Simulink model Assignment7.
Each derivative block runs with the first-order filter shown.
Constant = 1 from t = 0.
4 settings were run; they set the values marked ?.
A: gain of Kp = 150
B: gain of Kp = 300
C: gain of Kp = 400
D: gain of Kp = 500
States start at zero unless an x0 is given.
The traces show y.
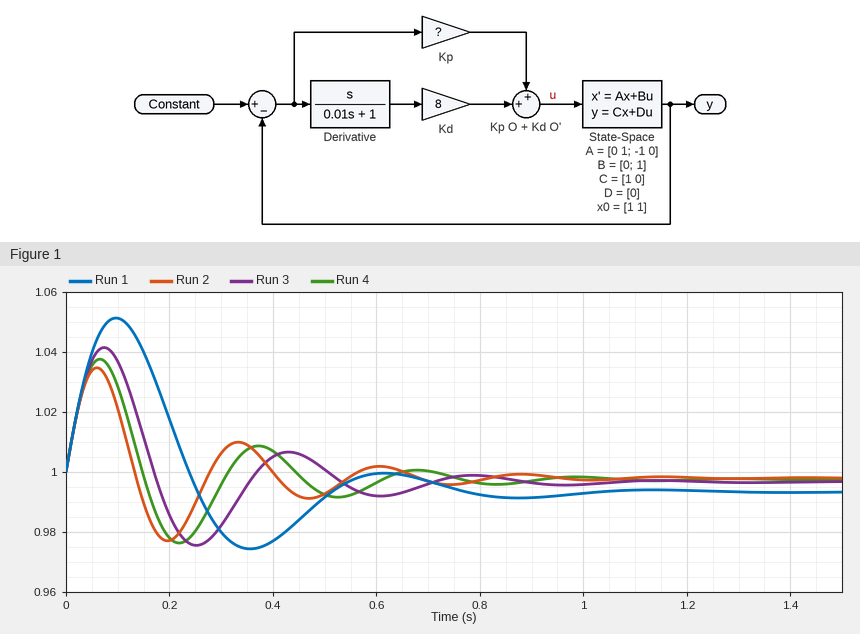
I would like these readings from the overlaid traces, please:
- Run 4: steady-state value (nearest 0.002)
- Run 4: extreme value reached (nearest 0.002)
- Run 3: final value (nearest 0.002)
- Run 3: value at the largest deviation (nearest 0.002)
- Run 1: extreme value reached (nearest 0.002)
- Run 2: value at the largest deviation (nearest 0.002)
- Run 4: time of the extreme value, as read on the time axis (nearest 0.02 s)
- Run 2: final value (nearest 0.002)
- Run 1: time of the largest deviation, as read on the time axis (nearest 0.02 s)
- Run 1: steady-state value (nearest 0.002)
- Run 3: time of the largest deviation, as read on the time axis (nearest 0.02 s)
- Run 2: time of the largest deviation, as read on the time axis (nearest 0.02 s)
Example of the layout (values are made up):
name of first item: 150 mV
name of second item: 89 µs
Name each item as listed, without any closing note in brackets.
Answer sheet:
Run 4: steady-state value: 0.998
Run 4: extreme value reached: 1.038
Run 3: final value: 0.996
Run 3: value at the largest deviation: 1.042
Run 1: extreme value reached: 1.052
Run 2: value at the largest deviation: 1.034
Run 4: time of the extreme value, as read on the time axis: 0.06 s
Run 2: final value: 0.998
Run 1: time of the largest deviation, as read on the time axis: 0.10 s
Run 1: steady-state value: 0.994
Run 3: time of the largest deviation, as read on the time axis: 0.08 s
Run 2: time of the largest deviation, as read on the time axis: 0.06 s
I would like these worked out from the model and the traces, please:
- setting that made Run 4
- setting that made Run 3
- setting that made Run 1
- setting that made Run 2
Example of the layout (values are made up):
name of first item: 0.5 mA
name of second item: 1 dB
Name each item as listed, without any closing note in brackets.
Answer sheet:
setting that made Run 4: C
setting that made Run 3: B
setting that made Run 1: A
setting that made Run 2: D
